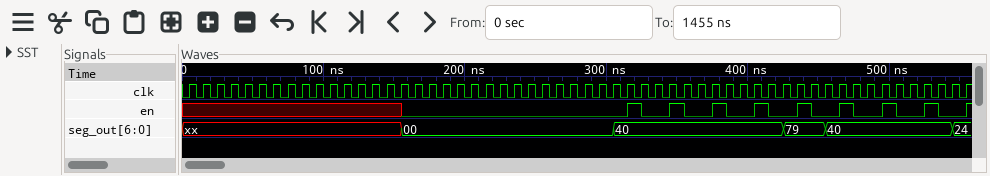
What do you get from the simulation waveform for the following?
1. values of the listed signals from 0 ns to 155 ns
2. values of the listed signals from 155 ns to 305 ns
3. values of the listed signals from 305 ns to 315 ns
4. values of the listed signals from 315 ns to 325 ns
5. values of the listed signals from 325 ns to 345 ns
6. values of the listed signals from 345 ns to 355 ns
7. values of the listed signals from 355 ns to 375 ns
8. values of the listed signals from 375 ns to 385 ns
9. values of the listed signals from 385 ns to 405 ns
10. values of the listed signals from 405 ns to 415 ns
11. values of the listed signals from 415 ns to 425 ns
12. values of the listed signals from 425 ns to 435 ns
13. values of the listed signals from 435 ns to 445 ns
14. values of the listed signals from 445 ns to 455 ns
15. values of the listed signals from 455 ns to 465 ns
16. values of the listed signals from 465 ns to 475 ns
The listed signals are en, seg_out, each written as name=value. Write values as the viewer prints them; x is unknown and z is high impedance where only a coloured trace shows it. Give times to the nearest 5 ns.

en=x, seg_out=xx
en=0, seg_out=00
en=0, seg_out=40
en=1, seg_out=40
en=0, seg_out=40
en=1, seg_out=40
en=0, seg_out=40
en=1, seg_out=40
en=0, seg_out=40
en=1, seg_out=40
en=0, seg_out=40
en=0, seg_out=79
en=1, seg_out=79
en=0, seg_out=79
en=0, seg_out=40
en=1, seg_out=40
